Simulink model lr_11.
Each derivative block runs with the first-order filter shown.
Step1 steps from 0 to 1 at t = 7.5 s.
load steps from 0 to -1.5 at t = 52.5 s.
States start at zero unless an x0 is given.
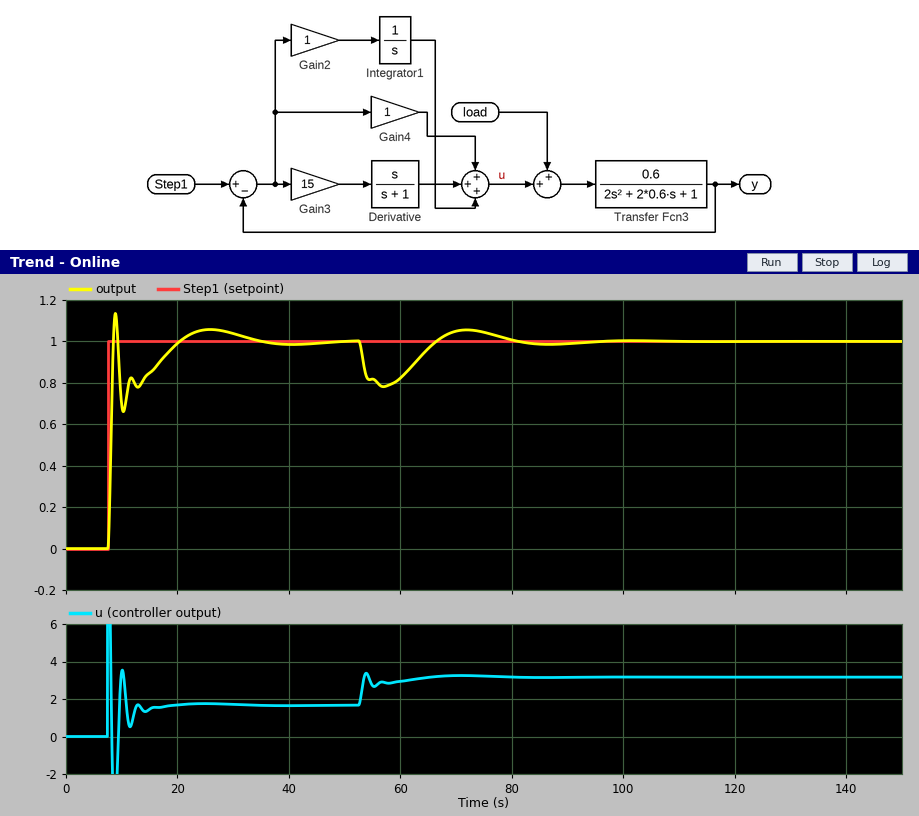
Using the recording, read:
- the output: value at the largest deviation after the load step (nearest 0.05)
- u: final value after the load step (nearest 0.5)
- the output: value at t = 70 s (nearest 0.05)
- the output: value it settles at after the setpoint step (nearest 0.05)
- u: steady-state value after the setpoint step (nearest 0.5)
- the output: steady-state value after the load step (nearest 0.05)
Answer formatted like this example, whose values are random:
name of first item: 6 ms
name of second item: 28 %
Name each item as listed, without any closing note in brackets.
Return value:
the output: value at the largest deviation after the load step: 0.80
u: final value after the load step: 3.0
the output: value at t = 70 s: 1.05
the output: value it settles at after the setpoint step: 1.00
u: steady-state value after the setpoint step: 1.5
the output: steady-state value after the load step: 1.00
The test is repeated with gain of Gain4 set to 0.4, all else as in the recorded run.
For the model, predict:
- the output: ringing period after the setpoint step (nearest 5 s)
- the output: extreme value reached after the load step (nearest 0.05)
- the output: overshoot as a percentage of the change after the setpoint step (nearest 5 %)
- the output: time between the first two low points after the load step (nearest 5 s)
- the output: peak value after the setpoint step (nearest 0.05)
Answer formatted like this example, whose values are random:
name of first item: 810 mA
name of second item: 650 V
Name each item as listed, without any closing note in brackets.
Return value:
the output: ringing period after the setpoint step: 15 s
the output: extreme value reached after the load step: 0.75
the output: overshoot as a percentage of the change after the setpoint step: 10 %
the output: time between the first two low points after the load step: 30 s
the output: peak value after the setpoint step: 1.10
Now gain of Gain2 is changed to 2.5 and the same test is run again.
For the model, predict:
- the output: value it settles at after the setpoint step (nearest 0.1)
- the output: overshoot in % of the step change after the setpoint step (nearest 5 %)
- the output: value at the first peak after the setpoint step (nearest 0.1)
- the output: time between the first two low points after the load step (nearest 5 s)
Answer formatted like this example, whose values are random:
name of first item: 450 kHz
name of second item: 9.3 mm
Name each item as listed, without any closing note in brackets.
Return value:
the output: value it settles at after the setpoint step: 1.0
the output: overshoot in % of the step change after the setpoint step: 20 %
the output: value at the first peak after the setpoint step: 1.2
the output: time between the first two low points after the load step: 20 s
